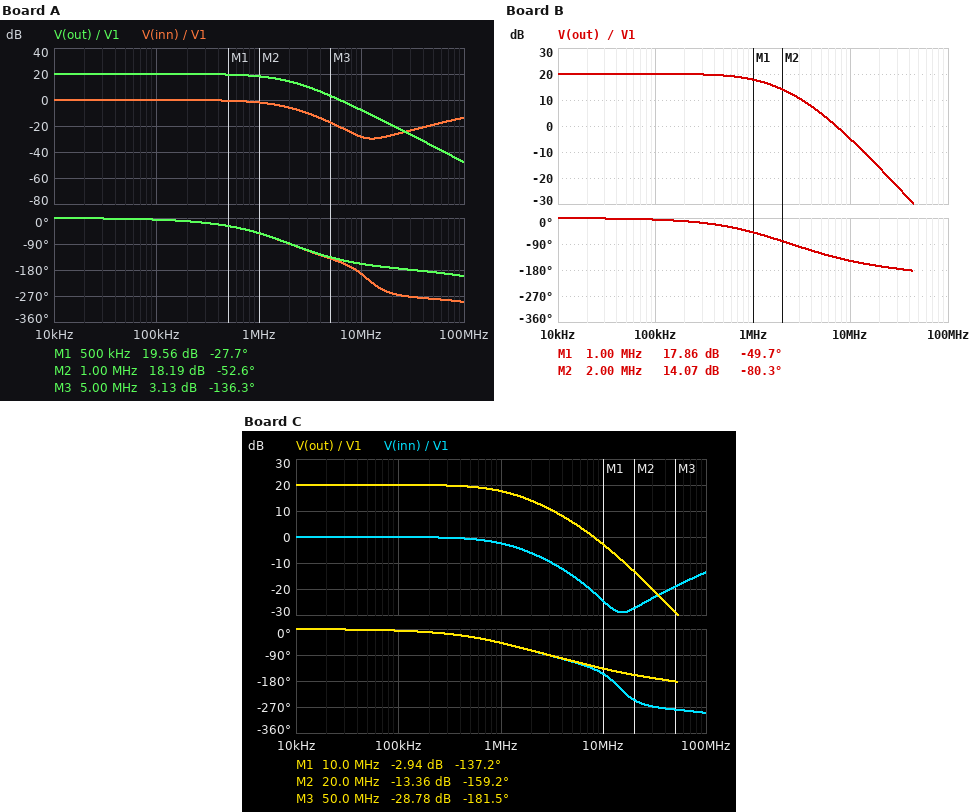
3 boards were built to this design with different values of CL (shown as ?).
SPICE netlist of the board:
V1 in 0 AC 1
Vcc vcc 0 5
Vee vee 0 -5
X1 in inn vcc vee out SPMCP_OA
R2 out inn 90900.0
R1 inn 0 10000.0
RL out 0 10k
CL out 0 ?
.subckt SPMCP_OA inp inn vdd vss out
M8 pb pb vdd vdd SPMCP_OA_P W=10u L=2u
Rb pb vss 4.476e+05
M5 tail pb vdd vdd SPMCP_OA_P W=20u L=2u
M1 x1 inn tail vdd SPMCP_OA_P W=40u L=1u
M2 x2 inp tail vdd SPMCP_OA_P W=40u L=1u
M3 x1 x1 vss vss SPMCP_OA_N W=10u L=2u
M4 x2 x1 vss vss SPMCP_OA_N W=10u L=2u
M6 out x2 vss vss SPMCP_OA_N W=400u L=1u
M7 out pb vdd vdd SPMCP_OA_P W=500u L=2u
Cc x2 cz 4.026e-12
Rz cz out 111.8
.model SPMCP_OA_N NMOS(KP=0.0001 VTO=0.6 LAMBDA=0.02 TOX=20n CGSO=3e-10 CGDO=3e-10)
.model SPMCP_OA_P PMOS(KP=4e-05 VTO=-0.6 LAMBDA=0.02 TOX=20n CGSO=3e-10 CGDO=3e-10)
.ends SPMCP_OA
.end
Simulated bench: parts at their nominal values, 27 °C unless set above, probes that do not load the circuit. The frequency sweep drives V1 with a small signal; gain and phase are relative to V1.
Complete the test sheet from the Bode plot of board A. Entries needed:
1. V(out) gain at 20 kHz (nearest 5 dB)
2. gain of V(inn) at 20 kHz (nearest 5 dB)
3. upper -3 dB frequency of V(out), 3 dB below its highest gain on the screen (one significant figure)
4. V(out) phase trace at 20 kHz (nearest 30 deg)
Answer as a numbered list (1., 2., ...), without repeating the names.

1. 20 dB
2. 0 dB
3. 1 MHz
4. 0 deg
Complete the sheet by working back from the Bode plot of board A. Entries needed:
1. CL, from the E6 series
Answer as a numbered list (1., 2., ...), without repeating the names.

1. 330 pF
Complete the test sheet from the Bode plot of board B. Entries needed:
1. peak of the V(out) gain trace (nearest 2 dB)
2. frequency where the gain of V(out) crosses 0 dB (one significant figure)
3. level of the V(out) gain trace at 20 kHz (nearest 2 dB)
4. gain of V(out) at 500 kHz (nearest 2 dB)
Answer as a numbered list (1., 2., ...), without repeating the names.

1. 20 dB
2. 7 MHz
3. 20 dB
4. 20 dB
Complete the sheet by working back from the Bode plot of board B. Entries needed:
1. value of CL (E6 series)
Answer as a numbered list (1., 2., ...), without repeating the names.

1. 220 pF
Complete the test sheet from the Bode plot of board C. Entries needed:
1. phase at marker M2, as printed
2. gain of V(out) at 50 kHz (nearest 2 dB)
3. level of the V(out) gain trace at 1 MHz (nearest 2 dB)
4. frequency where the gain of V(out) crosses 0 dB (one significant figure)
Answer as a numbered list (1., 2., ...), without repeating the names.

1. -159.2 deg
2. 20 dB
3. 18 dB
4. 8 MHz
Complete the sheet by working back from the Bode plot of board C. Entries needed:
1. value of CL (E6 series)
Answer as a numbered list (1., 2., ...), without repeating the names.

1. 150 pF
